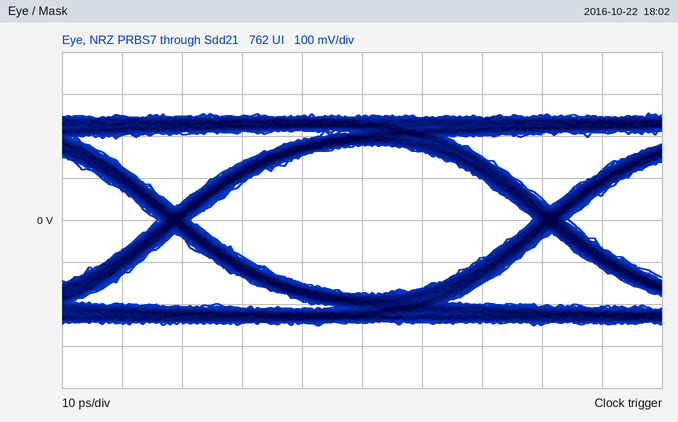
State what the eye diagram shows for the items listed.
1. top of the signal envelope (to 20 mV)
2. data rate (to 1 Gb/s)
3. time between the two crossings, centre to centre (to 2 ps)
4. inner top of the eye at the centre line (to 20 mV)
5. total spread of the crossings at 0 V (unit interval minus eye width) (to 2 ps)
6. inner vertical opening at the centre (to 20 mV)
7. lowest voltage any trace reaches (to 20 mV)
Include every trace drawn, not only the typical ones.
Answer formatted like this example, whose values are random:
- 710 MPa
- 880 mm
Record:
- 260 mV
- 16 Gb/s
- 62 ps
- 180 mV
- 6 ps
- 360 mV
- -260 mV
